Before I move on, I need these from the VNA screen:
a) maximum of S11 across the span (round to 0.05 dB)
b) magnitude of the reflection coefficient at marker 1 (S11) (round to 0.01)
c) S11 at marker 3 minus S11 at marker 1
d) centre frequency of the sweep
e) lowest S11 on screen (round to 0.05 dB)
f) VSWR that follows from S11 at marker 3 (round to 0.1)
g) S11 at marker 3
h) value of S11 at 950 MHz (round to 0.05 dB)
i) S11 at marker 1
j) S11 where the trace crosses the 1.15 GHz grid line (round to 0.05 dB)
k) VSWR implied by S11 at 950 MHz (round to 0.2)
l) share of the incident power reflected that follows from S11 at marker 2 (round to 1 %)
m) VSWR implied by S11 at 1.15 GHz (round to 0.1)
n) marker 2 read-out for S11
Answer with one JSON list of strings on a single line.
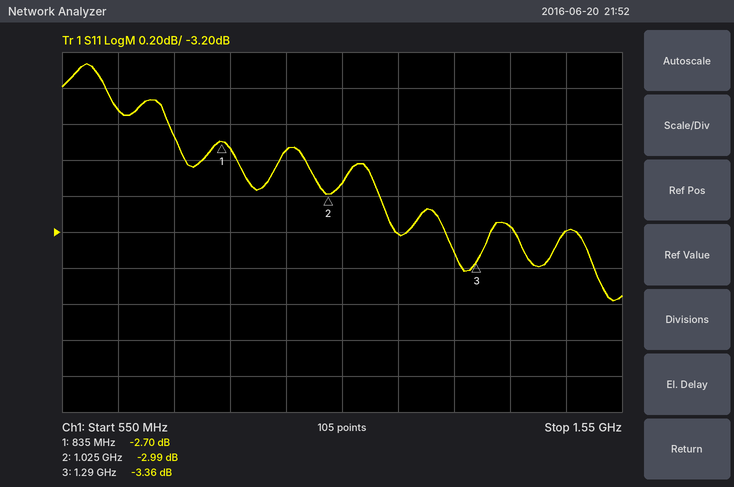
["-2.25 dB", "0.73", "-0.66 dB", "1.05 GHz", "-3.60 dB", "5.2", "-3.36 dB", "-2.75 dB", "-2.70 dB", "-3.20 dB", "6.4", "50 %", "5.5", "-2.99 dB"]
